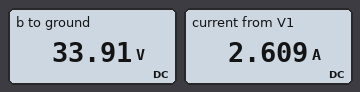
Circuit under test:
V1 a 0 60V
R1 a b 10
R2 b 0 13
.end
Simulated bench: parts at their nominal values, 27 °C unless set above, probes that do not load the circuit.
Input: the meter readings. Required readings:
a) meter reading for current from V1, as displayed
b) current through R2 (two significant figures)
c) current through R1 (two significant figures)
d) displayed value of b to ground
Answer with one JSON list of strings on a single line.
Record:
["2.609 A", "2.6 A", "2.6 A", "33.91 V"]
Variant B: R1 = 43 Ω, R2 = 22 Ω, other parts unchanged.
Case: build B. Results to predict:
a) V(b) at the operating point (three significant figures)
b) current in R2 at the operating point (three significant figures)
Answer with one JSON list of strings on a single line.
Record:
["20.3 V", "923 mA"]
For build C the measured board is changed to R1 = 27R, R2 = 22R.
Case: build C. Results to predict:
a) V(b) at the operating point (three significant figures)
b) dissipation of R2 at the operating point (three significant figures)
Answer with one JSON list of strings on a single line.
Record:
["26.9 V", "33.0 W"]
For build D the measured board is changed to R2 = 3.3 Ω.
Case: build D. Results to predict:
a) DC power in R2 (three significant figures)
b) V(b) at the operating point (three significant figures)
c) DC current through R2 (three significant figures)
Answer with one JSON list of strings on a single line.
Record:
["67.2 W", "14.9 V", "4.51 A"]
